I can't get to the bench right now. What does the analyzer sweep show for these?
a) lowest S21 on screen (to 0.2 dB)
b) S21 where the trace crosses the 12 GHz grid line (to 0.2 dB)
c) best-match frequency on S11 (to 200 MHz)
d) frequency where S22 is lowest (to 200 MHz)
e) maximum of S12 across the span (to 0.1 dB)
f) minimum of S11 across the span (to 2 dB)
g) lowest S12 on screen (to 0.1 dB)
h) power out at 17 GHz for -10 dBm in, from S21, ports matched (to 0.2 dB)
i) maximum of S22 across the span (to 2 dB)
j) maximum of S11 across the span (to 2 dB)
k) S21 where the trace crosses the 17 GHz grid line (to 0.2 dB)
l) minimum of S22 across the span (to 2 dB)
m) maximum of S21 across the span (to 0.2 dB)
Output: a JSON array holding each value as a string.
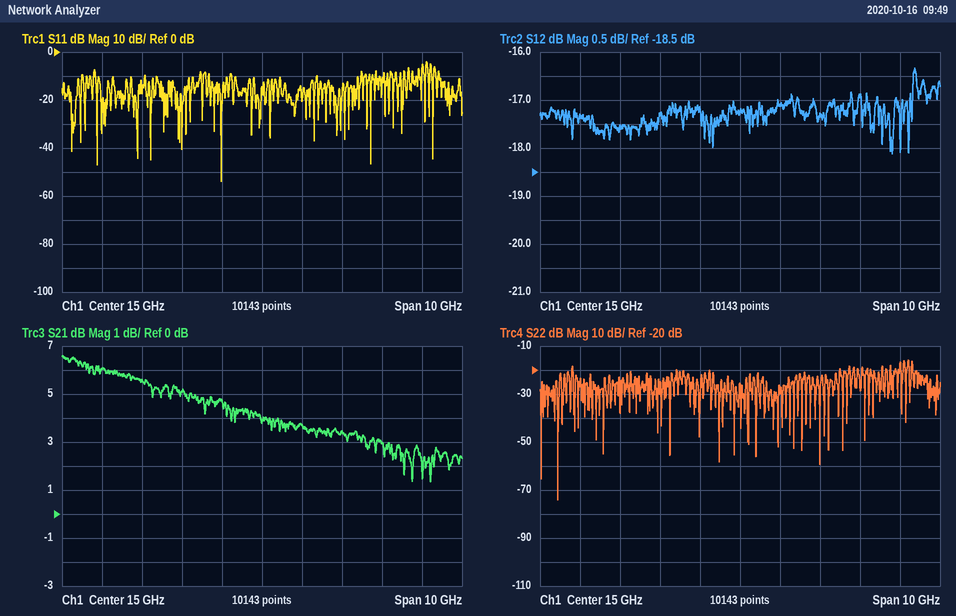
["1.4 dB", "5.6 dB", "14.0 GHz", "10.4 GHz", "-16.3 dB", "-54 dB", "-18.1 dB", "-6.6 dBm", "-16 dB", "-4 dB", "3.4 dB", "-74 dB", "6.6 dB"]
